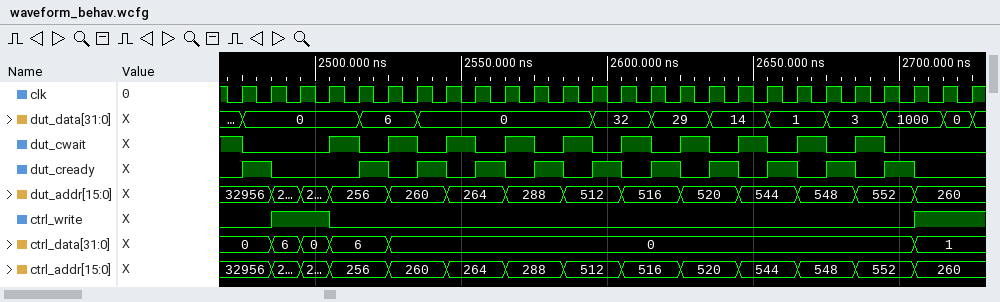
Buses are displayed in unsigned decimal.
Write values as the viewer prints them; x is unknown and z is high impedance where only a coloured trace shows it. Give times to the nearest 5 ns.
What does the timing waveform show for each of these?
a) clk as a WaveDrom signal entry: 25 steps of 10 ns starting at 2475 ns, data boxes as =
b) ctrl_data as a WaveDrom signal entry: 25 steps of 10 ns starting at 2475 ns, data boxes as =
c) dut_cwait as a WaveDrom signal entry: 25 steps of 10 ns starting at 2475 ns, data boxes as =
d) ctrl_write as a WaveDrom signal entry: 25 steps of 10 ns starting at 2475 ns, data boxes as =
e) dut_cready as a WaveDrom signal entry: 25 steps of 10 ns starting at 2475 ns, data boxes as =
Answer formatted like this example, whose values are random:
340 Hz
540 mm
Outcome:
{name: 'clk', wave: 'p........................'}
{name: 'ctrl_data', wave: '====.=.................=.', data: '0 6 0 6 0 1'}
{name: 'dut_cwait', wave: '0..10101010101010101010..'}
{name: 'ctrl_write', wave: '01.0...................1.'}
{name: 'dut_cready', wave: '10..10101010101010101010.'}
